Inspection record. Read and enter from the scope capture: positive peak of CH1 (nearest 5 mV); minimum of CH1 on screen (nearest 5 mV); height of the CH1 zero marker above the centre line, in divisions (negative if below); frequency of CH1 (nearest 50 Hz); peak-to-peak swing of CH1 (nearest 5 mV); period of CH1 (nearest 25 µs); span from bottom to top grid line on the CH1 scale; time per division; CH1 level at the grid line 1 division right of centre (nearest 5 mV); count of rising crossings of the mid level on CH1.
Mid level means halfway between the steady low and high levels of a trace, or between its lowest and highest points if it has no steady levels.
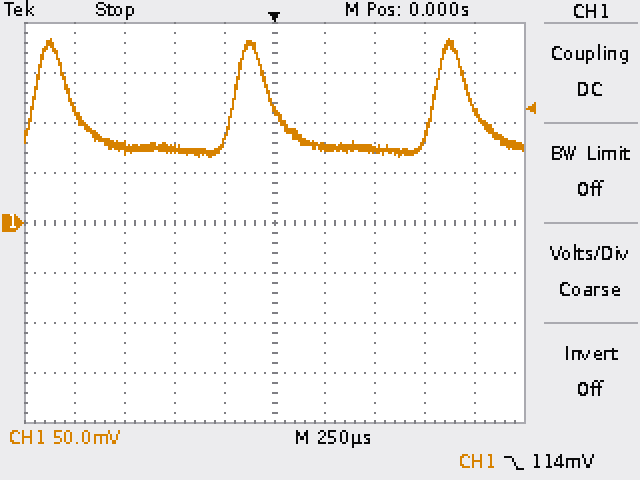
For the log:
185 mV
65 mV
0.0 div
1.00 kHz
120 mV
1.000 ms
400 mV
250 µs
75 mV
3
